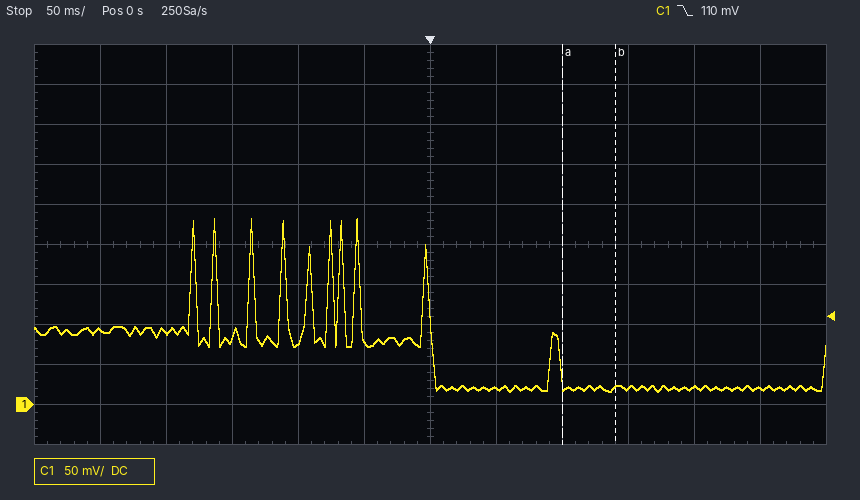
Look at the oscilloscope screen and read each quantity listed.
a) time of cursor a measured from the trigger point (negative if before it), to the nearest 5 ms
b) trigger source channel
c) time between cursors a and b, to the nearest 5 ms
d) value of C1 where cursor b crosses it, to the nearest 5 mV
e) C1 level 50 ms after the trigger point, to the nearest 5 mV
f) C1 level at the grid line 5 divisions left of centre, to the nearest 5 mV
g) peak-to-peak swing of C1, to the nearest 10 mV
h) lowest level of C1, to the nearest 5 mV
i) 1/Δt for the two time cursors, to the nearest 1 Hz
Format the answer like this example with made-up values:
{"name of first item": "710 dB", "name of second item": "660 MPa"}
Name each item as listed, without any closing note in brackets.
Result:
{"time of cursor a measured from the trigger point (negative if before it), to the nearest 5 ms": "+100 ms", "trigger source channel": "C1", "time between cursors a and b, to the nearest 5 ms": "40 ms", "value of C1 where cursor b crosses it, to the nearest 5 mV": "20 mV", "C1 level 50 ms after the trigger point, to the nearest 5 mV": "20 mV", "C1 level at the grid line 5 divisions left of centre, to the nearest 5 mV": "95 mV", "peak-to-peak swing of C1, to the nearest 10 mV": "220 mV", "lowest level of C1, to the nearest 5 mV": "15 mV", "1/Δt for the two time cursors, to the nearest 1 Hz": "25 Hz"}
